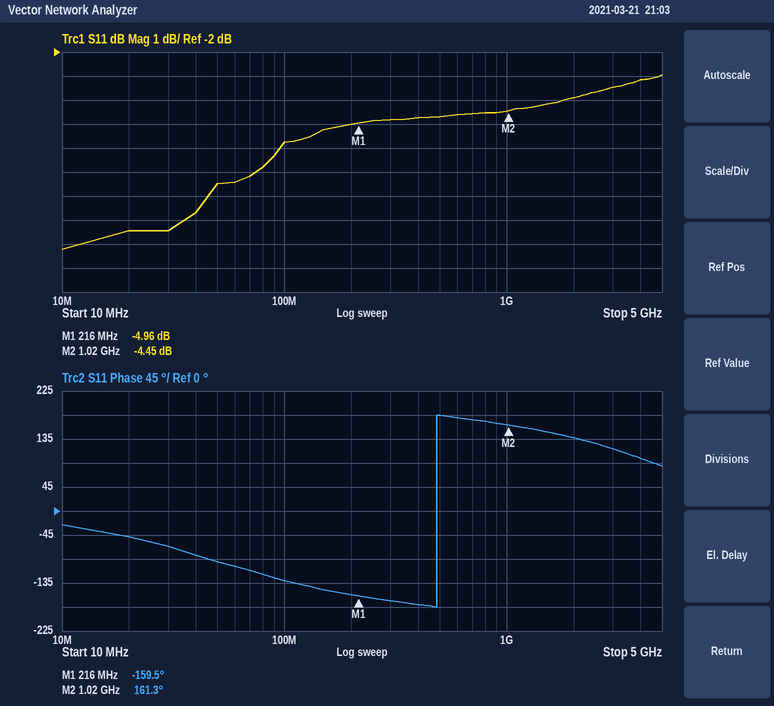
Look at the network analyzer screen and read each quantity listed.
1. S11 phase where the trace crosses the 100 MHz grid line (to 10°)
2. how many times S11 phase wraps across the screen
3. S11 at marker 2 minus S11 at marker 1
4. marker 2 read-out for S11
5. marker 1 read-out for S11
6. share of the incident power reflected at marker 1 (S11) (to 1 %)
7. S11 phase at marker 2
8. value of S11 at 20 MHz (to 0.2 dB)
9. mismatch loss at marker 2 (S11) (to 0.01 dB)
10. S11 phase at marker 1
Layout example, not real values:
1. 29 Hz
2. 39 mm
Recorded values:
1. -130°
2. 1
3. 0.51 dB
4. -4.45 dB
5. -4.96 dB
6. 32 %
7. 161.3°
8. -9.4 dB
9. 1.93 dB
10. -159.5°
